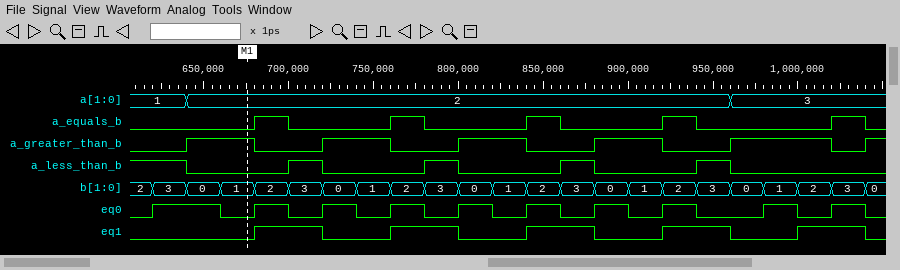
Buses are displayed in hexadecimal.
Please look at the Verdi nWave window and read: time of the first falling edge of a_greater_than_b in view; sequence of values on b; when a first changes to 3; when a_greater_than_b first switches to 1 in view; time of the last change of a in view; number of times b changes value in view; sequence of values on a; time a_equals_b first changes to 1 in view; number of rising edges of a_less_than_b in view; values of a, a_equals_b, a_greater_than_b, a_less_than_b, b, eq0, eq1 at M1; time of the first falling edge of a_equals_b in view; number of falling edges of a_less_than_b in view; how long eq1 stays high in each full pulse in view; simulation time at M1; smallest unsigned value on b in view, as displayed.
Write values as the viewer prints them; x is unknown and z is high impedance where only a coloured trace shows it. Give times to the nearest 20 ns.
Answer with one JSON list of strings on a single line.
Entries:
["680 ns", "2, 3, 0, 1, 2, 3, 0, 1, 2, 3, 0, 1, 2, 3, 0, 1, 2, 3, 0, 1, 2, 3, 0", "960 ns", "640 ns", "960 ns", "22", "1, 2, 3", "680 ns", "4", "a=2, a_equals_b=0, a_greater_than_b=1, a_less_than_b=0, b=1, eq0=0, eq1=0", "700 ns", "5", "40 ns, 40 ns, 40 ns, 40 ns, 40 ns", "680 ns", "0"]
